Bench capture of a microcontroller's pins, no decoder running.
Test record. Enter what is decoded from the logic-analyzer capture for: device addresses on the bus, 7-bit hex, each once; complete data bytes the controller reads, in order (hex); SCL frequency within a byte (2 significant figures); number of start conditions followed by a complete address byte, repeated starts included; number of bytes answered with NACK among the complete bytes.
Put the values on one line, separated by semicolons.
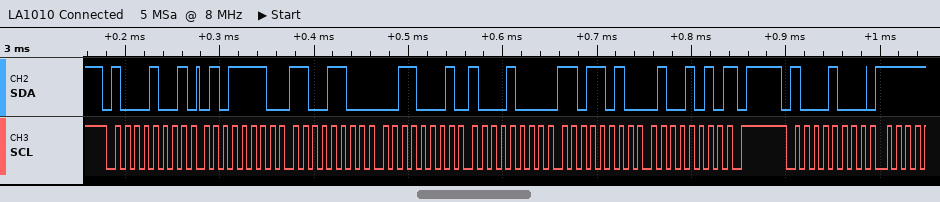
0x44; 5E CC 31 88 DA 4A; 100 kHz; 2; 1
